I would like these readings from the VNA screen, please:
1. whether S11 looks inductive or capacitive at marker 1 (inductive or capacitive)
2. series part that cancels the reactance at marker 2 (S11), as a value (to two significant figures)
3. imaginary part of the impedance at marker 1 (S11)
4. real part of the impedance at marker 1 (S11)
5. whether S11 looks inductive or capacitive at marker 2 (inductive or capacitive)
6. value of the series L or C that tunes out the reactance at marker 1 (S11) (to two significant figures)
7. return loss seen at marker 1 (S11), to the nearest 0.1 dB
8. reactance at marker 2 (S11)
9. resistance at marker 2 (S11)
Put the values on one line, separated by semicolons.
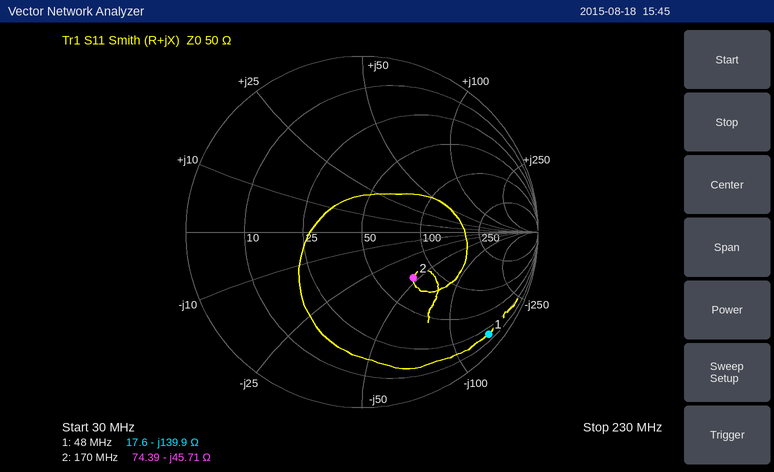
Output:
capacitive; 43 nH; -139.9 Ω; 17.6 Ω; capacitive; 460 nH; 0.7 dB; -45.71 Ω; 74.39 Ω
